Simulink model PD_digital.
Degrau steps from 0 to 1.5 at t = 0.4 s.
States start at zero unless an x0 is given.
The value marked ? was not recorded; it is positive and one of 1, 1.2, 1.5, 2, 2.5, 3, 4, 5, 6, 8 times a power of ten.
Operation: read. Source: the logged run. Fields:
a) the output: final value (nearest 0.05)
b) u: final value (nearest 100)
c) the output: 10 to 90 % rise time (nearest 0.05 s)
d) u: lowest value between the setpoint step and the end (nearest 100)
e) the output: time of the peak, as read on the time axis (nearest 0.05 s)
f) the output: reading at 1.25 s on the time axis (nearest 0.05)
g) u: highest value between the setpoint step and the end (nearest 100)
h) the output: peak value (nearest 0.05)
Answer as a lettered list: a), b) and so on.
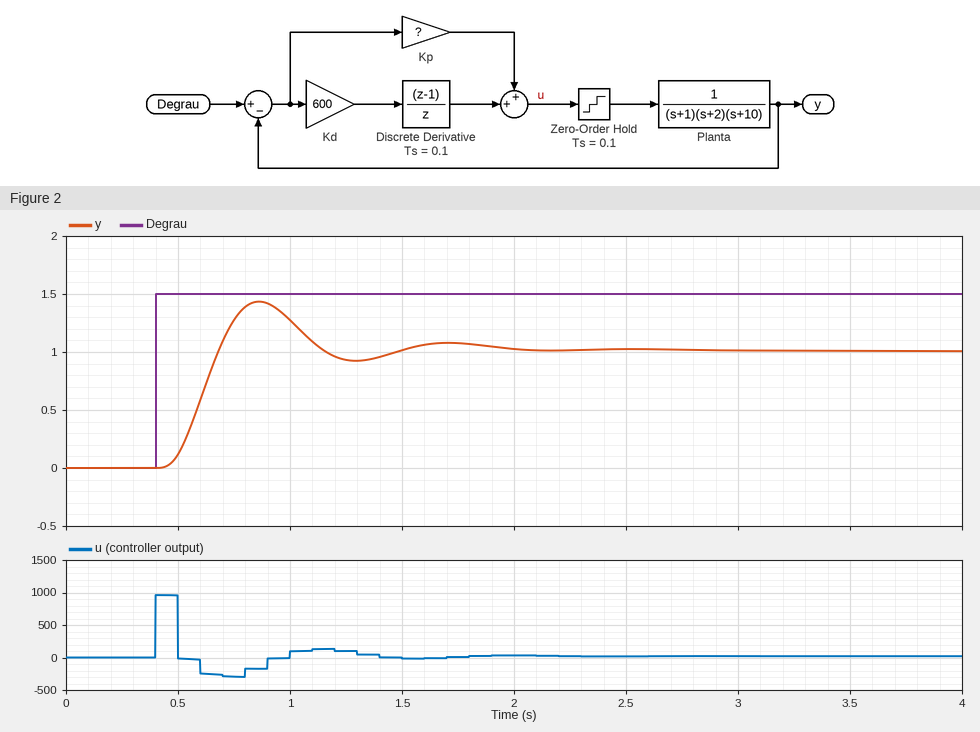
a) 1.00
b) 0
c) 0.15 s
d) -300
e) 0.85 s
f) 0.95
g) 1000
h) 1.45
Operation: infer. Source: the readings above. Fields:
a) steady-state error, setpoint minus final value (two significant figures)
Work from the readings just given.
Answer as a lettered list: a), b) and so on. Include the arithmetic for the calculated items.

a) 1.5 - 1 = 0.50
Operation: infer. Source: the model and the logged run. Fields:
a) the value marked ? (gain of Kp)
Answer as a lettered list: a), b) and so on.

a) 40
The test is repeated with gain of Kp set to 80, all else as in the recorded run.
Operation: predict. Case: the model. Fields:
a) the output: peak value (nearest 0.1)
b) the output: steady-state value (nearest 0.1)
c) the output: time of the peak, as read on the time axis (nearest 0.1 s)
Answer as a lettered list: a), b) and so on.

a) 1.6
b) 1.2
c) 0.9 s
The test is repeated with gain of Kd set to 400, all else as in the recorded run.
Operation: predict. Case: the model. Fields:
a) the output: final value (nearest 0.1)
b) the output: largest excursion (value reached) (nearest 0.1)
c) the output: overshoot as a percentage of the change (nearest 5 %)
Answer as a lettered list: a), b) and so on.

a) 1.0
b) 1.2
c) 20 %
